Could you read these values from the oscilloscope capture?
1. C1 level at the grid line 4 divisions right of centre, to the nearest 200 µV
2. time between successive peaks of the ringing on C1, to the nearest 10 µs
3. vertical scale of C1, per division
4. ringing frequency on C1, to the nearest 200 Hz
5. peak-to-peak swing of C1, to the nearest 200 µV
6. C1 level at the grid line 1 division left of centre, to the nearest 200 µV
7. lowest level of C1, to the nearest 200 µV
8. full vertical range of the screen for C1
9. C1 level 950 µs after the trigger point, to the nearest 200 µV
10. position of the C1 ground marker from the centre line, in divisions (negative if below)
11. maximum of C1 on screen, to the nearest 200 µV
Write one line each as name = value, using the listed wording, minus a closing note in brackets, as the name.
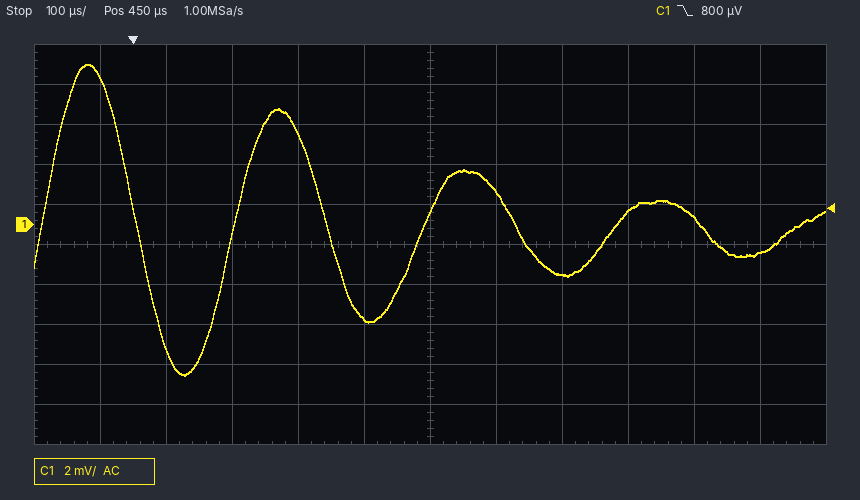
C1 level at the grid line 4 divisions right of centre, to the nearest 200 µV = 400 µV
time between successive peaks of the ringing on C1, to the nearest 10 µs = 290 µs
vertical scale of C1, per division = 2 mV
ringing frequency on C1, to the nearest 200 Hz = 3.4 kHz
peak-to-peak swing of C1, to the nearest 200 µV = 15.6 mV
C1 level at the grid line 1 division left of centre, to the nearest 200 µV = -4.8 mV
lowest level of C1, to the nearest 200 µV = -7.6 mV
full vertical range of the screen for C1 = 20 mV
C1 level 950 µs after the trigger point, to the nearest 200 µV = -1.4 mV
position of the C1 ground marker from the centre line, in divisions = +0.5 div
maximum of C1 on screen, to the nearest 200 µV = 8.0 mV
